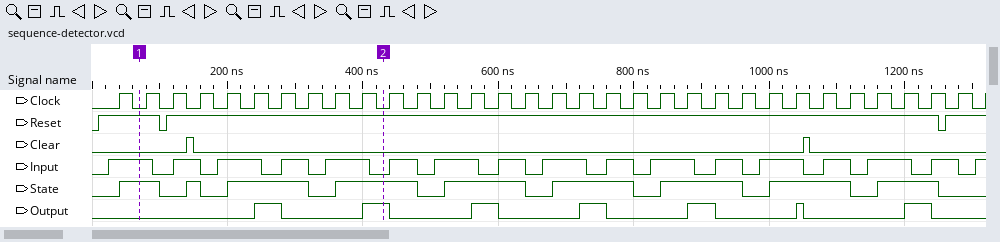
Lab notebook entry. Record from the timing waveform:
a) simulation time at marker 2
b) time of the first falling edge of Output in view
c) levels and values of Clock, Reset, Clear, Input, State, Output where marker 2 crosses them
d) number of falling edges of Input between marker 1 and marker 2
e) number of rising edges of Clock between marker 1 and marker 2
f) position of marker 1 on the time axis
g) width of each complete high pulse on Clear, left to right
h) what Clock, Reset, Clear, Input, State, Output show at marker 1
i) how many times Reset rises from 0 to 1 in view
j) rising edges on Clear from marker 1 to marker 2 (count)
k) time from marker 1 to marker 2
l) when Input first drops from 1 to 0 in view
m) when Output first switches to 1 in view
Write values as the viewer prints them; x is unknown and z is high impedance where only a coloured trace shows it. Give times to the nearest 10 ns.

430 ns
280 ns
Clock=0, Reset=1, Clear=0, Input=0, State=1, Output=1
5
9
70 ns
10 ns, 10 ns
Clock=0, Reset=1, Clear=0, Input=1, State=1, Output=0
3
1
360 ns
90 ns
240 ns
